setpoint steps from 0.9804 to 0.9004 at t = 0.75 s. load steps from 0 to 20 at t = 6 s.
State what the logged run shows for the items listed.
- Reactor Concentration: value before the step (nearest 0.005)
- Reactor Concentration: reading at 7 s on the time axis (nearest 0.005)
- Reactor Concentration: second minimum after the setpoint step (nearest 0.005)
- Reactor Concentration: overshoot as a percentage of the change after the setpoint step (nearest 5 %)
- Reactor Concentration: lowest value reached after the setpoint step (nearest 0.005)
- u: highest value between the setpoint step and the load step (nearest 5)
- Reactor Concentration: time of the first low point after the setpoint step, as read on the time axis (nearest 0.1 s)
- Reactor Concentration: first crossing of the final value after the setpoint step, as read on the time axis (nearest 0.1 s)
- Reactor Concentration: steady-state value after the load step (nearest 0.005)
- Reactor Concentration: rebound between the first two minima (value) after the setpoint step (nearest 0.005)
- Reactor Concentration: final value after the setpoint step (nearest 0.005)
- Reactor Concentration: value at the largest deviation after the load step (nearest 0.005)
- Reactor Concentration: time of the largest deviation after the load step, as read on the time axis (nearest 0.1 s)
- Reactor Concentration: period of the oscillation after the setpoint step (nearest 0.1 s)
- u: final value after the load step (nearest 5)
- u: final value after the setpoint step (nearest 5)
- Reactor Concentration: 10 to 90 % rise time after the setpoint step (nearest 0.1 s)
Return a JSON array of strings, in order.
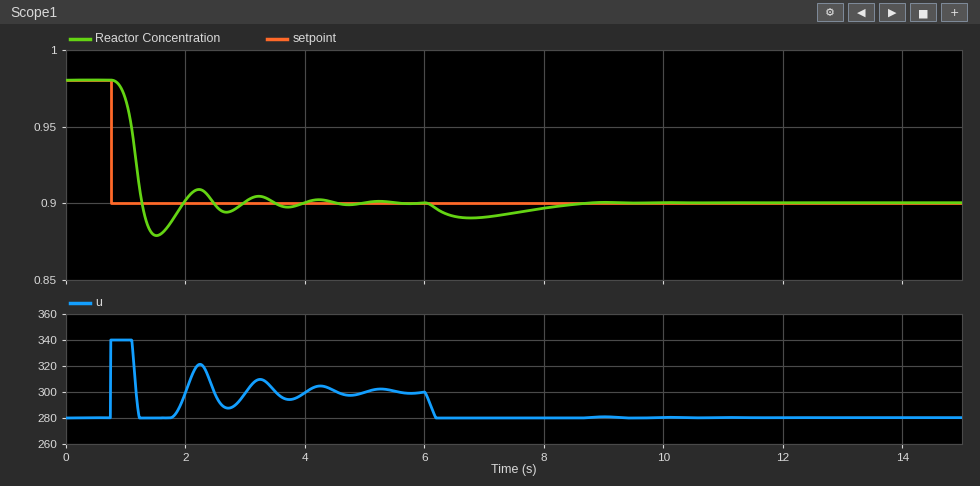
["0.980", "0.890", "0.895", "25 %", "0.880", "340", "1.5 s", "1.3 s", "0.900", "0.910", "0.900", "0.890", "6.8 s", "1.2 s", "280", "300", "0.3 s"]
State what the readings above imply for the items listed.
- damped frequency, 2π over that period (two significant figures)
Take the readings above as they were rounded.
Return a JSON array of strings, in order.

["5.2 rad/s"]
